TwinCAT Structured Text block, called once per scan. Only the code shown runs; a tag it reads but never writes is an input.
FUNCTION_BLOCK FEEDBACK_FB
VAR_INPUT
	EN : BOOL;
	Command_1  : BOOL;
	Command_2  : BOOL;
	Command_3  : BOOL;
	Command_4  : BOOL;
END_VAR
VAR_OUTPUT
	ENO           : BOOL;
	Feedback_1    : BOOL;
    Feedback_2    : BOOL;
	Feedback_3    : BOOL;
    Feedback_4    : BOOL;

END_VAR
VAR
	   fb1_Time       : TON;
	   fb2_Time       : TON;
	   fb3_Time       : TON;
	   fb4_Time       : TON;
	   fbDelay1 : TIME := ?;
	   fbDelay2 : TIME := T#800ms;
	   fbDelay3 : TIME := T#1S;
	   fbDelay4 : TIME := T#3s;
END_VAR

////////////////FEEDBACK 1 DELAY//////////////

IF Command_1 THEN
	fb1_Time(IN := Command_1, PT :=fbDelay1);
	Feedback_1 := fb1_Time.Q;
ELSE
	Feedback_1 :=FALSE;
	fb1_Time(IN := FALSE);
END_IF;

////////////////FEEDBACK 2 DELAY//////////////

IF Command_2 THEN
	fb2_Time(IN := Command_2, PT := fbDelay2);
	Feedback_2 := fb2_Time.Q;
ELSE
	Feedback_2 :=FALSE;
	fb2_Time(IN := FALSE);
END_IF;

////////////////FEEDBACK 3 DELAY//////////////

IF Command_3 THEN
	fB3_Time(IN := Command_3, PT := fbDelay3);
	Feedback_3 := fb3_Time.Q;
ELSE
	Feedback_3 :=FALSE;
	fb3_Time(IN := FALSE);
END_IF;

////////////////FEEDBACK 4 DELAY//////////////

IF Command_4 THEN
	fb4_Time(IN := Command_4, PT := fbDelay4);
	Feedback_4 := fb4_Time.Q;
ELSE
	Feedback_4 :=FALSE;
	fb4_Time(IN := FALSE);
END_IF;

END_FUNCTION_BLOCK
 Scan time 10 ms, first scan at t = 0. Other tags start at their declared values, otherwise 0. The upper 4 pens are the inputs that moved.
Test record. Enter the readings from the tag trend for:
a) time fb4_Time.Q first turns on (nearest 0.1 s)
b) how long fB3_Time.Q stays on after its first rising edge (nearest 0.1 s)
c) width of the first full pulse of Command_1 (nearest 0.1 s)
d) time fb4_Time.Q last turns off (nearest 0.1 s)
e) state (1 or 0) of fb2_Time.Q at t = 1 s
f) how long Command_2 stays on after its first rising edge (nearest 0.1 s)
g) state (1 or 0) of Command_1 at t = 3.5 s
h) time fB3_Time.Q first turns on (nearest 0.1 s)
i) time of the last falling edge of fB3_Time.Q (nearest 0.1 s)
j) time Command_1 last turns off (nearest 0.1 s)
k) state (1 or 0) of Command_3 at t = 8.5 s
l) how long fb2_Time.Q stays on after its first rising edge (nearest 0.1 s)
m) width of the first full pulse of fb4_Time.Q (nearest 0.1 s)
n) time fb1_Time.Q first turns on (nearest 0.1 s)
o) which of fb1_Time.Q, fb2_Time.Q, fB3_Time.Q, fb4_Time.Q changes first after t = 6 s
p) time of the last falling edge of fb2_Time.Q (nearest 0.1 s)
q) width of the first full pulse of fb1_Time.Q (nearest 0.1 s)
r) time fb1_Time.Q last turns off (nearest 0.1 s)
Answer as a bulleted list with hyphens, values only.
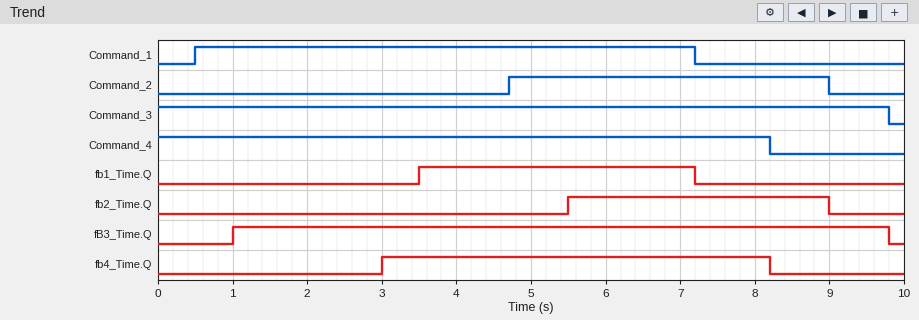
- 3.0 s
- 8.8 s
- 6.7 s
- 8.2 s
- 0
- 4.3 s
- 1
- 1.0 s
- 9.8 s
- 7.2 s
- 1
- 3.5 s
- 5.2 s
- 3.5 s
- fb1_Time.Q
- 9.0 s
- 3.7 s
- 7.2 s
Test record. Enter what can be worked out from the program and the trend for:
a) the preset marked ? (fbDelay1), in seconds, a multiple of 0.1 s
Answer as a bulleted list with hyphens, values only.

- 3.0 s
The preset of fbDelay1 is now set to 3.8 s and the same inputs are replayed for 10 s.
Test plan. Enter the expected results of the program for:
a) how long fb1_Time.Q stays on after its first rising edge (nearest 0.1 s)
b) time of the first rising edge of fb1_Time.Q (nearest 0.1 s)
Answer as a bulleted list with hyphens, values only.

- 2.9 s
- 4.3 s
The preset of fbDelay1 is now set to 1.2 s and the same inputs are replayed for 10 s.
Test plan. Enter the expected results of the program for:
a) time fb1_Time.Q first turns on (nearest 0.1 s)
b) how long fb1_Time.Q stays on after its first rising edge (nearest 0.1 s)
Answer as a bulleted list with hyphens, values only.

- 1.7 s
- 5.5 s
